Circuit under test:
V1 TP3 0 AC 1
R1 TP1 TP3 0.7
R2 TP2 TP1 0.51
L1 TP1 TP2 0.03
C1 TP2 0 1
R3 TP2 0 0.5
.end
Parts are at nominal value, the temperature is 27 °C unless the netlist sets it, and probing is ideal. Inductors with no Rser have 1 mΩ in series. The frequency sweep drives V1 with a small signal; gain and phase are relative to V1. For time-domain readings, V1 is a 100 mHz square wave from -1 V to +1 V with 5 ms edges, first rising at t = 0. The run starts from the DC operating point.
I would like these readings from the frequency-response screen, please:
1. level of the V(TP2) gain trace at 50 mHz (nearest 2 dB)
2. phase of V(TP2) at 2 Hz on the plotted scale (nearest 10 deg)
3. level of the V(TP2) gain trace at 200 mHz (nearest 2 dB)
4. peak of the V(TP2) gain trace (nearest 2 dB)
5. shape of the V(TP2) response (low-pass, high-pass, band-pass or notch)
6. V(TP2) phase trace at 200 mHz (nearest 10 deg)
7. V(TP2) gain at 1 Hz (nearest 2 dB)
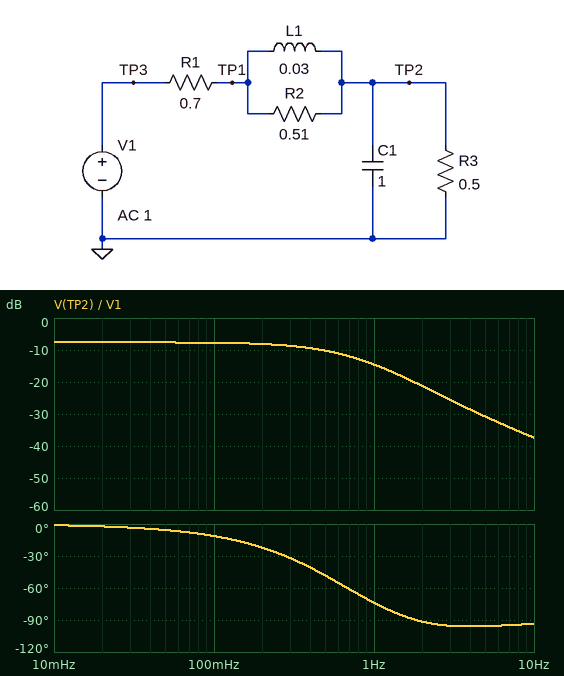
-8 dB
-90 deg
-8 dB
-8 dB
low-pass
-20 deg
-14 dB
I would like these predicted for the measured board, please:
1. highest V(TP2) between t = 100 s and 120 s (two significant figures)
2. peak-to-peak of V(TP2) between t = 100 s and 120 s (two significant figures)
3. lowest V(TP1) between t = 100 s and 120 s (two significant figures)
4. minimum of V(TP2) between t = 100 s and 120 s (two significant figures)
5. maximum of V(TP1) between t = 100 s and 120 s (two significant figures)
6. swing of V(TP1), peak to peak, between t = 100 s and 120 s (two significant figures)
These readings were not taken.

420 mV
830 mV
-420 mV
-420 mV
420 mV
830 mV
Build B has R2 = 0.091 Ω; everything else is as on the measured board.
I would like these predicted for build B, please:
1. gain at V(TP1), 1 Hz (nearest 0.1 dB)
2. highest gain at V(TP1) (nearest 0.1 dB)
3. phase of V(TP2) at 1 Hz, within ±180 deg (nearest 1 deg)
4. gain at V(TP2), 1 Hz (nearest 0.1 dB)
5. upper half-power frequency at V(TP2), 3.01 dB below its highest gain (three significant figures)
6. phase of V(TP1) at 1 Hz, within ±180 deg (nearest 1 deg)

-14.2 dB
-7.6 dB
-65 deg
-14.7 dB
503 mHz
-35 deg
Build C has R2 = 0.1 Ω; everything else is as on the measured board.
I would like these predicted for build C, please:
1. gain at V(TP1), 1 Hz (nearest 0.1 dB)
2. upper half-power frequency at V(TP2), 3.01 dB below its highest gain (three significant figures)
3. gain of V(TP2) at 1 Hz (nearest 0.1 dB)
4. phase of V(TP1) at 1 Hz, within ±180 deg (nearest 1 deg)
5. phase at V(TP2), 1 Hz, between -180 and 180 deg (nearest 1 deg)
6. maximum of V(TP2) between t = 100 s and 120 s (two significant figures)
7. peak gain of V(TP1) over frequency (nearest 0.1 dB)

-14.2 dB
504 mHz
-14.8 dB
-33 deg
-65 deg
420 mV
-7.6 dB
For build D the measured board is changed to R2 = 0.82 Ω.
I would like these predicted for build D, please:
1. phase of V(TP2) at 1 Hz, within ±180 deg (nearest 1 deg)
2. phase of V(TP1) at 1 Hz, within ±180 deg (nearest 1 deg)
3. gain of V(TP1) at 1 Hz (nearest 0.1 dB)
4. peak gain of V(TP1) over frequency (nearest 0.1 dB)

-75 deg
19 deg
-18.4 dB
-5.4 dB
